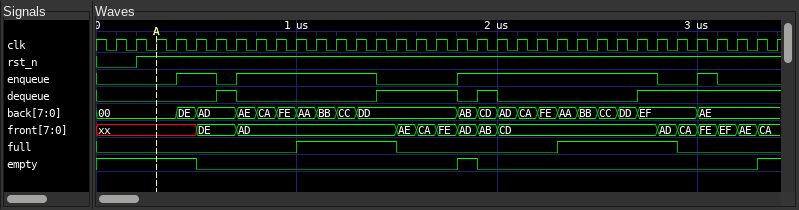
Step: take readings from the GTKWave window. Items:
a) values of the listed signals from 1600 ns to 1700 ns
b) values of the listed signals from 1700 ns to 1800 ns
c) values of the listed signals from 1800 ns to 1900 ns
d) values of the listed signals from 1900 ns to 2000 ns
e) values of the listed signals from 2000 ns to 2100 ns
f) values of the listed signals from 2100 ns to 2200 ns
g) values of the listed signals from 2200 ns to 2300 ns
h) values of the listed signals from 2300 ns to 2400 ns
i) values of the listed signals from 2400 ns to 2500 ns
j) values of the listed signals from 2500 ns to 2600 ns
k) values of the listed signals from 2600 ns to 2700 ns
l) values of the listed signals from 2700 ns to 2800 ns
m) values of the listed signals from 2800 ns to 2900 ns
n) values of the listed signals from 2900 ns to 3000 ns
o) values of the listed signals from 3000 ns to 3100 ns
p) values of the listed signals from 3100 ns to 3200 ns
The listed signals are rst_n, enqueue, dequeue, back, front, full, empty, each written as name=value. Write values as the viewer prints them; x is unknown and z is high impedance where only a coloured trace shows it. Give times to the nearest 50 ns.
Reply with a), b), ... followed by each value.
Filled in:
a) rst_n=1, enqueue=0, dequeue=1, back=DD, front=CA, full=0, empty=0
b) rst_n=1, enqueue=0, dequeue=1, back=DD, front=FE, full=0, empty=0
c) rst_n=1, enqueue=1, dequeue=0, back=AB, front=AD, full=0, empty=1
d) rst_n=1, enqueue=1, dequeue=1, back=CD, front=AB, full=0, empty=0
e) rst_n=1, enqueue=1, dequeue=0, back=AD, front=CD, full=0, empty=0
f) rst_n=1, enqueue=1, dequeue=0, back=CA, front=CD, full=0, empty=0
g) rst_n=1, enqueue=1, dequeue=0, back=FE, front=CD, full=0, empty=0
h) rst_n=1, enqueue=1, dequeue=0, back=AA, front=CD, full=1, empty=0
i) rst_n=1, enqueue=1, dequeue=0, back=BB, front=CD, full=1, empty=0
j) rst_n=1, enqueue=1, dequeue=0, back=CC, front=CD, full=1, empty=0
k) rst_n=1, enqueue=1, dequeue=0, back=DD, front=CD, full=1, empty=0
l) rst_n=1, enqueue=1, dequeue=1, back=EF, front=CD, full=1, empty=0
m) rst_n=1, enqueue=0, dequeue=1, back=EF, front=AD, full=1, empty=0
n) rst_n=1, enqueue=0, dequeue=1, back=EF, front=CA, full=0, empty=0
o) rst_n=1, enqueue=1, dequeue=1, back=AE, front=FE, full=0, empty=0
p) rst_n=1, enqueue=0, dequeue=1, back=AE, front=EF, full=0, empty=0
